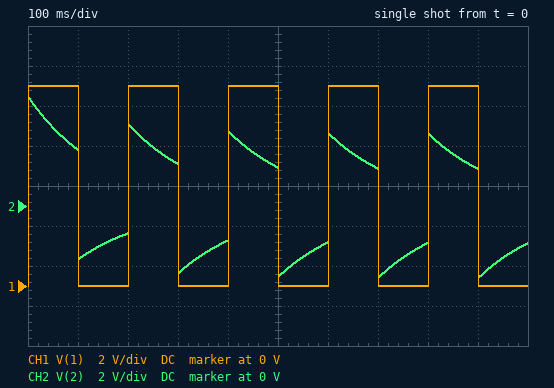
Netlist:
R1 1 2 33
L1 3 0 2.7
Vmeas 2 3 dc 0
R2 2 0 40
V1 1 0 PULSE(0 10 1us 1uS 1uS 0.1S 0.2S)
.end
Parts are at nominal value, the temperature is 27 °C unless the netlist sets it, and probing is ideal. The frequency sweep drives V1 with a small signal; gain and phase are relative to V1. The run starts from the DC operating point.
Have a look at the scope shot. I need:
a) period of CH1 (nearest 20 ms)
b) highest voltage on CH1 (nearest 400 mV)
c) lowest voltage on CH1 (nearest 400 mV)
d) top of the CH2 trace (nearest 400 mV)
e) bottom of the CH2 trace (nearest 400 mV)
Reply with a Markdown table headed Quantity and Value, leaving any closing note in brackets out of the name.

| Quantity | Value |
|---|---|
| period of CH1 | 200 ms |
| highest voltage on CH1 | 10.0 V |
| lowest voltage on CH1 | 0 V |
| top of the CH2 trace | 5.6 V |
| bottom of the CH2 trace | -3.6 V |
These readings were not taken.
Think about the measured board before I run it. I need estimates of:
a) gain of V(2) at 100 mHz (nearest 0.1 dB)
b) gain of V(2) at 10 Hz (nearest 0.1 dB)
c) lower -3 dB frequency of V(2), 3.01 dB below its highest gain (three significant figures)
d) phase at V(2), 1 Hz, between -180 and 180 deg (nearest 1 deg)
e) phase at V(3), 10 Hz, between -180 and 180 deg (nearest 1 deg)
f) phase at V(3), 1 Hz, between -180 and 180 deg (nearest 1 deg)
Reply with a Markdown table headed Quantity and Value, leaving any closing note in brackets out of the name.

| Quantity | Value |
|---|---|
| gain of V(2) at 100 mHz | -25.8 dB |
| gain of V(2) at 10 Hz | -5.3 dB |
| lower -3 dB frequency of V(2), 3.01 dB below its highest gain | 1.07 Hz |
| phase at V(2), 1 Hz, between -180 and 180 deg | 47 deg |
| phase at V(3), 10 Hz, between -180 and 180 deg | 6 deg |
| phase at V(3), 1 Hz, between -180 and 180 deg | 47 deg |
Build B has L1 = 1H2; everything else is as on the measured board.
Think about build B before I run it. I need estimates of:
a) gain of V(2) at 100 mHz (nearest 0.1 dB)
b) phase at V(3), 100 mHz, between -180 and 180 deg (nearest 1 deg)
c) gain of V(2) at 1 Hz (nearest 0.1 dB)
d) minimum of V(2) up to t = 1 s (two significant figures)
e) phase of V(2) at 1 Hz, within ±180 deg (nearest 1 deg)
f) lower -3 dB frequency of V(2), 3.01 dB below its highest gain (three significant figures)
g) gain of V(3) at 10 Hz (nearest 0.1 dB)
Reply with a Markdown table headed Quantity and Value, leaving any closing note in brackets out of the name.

| Quantity | Value |
|---|---|
| gain of V(2) at 100 mHz | -32.8 dB |
| phase at V(3), 100 mHz, between -180 and 180 deg | 88 deg |
| gain of V(2) at 1 Hz | -13.5 dB |
| minimum of V(2) up to t = 1 s | -4.5 V |
| phase of V(2) at 1 Hz, within ±180 deg | 67 deg |
| lower -3 dB frequency of V(2), 3.01 dB below its highest gain | 2.40 Hz |
| gain of V(3) at 10 Hz | -5.5 dB |
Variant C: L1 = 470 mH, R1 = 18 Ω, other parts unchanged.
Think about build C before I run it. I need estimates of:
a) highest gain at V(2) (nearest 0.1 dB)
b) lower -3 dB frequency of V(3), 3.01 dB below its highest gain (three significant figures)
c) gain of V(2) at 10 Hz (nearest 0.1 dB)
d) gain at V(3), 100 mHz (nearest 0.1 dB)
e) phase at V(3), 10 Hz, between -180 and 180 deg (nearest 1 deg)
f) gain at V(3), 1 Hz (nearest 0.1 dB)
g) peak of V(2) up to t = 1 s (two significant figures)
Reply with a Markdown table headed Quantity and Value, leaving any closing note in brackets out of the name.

| Quantity | Value |
|---|---|
| highest gain at V(2) | -3.2 dB |
| lower -3 dB frequency of V(3), 3.01 dB below its highest gain | 4.20 Hz |
| gain of V(2) at 10 Hz | -3.9 dB |
| gain at V(3), 100 mHz | -35.7 dB |
| phase at V(3), 10 Hz, between -180 and 180 deg | 23 deg |
| gain at V(3), 1 Hz | -15.9 dB |
| peak of V(2) up to t = 1 s | 6.9 V |
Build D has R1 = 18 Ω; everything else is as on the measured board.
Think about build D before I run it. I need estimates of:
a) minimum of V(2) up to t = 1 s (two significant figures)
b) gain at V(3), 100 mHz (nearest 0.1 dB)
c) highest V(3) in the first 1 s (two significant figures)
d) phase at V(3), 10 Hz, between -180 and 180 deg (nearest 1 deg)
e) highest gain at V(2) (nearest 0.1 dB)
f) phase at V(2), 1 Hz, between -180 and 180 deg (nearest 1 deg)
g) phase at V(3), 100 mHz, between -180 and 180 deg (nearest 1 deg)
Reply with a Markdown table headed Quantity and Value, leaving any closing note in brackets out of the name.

| Quantity | Value |
|---|---|
| minimum of V(2) up to t = 1 s | -4.2 V |
| gain at V(3), 100 mHz | -20.6 dB |
| highest V(3) in the first 1 s | 6.9 V |
| phase at V(3), 10 Hz, between -180 and 180 deg | 4 deg |
| highest gain at V(2) | -3.2 dB |
| phase at V(2), 1 Hz, between -180 and 180 deg | 36 deg |
| phase at V(3), 100 mHz, between -180 and 180 deg | 82 deg |
